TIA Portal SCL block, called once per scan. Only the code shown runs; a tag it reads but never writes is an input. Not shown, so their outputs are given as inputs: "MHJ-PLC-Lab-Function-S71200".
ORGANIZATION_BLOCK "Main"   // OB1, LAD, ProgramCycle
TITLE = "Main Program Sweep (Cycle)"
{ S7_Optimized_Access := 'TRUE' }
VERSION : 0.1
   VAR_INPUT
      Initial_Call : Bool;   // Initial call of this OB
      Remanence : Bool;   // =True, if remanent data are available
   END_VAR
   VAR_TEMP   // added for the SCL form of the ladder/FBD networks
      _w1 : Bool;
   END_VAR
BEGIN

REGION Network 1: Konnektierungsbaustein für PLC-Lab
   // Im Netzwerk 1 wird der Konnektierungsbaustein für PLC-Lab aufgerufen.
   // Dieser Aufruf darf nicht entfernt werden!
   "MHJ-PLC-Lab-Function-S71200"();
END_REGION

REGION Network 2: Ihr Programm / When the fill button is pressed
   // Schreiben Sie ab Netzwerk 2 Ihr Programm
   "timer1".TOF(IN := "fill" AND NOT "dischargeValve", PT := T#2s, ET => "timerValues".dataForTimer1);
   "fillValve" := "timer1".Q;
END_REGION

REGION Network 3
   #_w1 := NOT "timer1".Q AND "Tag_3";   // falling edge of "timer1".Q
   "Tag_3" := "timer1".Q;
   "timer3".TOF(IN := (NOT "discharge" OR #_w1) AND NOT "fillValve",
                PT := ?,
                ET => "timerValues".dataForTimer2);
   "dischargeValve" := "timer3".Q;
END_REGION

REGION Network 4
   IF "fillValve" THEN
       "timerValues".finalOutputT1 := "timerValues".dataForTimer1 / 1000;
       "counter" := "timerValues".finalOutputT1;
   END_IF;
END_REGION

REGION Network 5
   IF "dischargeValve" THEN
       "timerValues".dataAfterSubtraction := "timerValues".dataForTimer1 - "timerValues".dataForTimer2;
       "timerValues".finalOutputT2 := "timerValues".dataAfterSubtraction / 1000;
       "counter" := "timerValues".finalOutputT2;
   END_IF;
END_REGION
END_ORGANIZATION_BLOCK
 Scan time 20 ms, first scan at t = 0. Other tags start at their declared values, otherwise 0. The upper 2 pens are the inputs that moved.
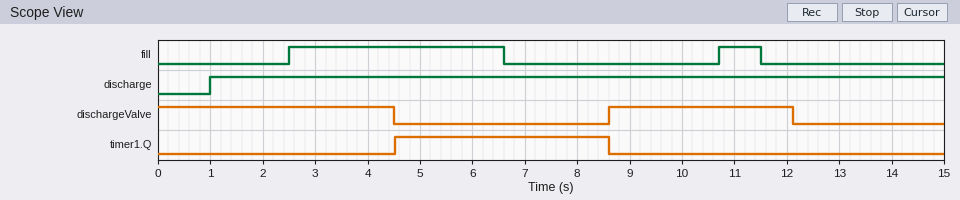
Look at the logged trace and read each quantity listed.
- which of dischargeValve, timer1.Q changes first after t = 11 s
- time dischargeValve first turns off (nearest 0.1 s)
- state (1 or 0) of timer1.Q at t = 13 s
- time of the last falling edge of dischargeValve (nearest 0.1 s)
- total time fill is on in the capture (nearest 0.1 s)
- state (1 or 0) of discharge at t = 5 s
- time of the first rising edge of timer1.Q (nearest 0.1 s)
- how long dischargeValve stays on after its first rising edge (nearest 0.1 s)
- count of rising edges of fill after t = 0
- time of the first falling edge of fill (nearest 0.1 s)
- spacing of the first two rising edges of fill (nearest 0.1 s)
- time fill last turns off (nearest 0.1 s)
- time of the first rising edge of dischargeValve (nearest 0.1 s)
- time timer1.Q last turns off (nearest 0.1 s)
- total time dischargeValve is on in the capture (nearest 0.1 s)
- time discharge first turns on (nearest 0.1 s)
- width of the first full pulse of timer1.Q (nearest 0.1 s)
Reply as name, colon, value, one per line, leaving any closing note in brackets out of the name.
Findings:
which of dischargeValve, timer1.Q changes first after t = 11 s: dischargeValve
time dischargeValve first turns off: 4.5 s
state (1 or 0) of timer1.Q at t = 13 s: 0
time of the last falling edge of dischargeValve: 12.1 s
total time fill is on in the capture: 4.9 s
state (1 or 0) of discharge at t = 5 s: 1
time of the first rising edge of timer1.Q: 4.5 s
how long dischargeValve stays on after its first rising edge: 3.5 s
count of rising edges of fill after t = 0: 2
time of the first falling edge of fill: 6.6 s
spacing of the first two rising edges of fill: 8.2 s
time fill last turns off: 11.5 s
time of the first rising edge of dischargeValve: 8.6 s
time timer1.Q last turns off: 8.6 s
total time dischargeValve is on in the capture: 8.0 s
time discharge first turns on: 1.0 s
width of the first full pulse of timer1.Q: 4.1 s
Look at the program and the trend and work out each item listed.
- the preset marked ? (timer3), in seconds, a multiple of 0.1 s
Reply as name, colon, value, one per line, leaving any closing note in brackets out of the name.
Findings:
the preset marked ? (timer3), in seconds, a multiple of 0.1 s: 3.5 s
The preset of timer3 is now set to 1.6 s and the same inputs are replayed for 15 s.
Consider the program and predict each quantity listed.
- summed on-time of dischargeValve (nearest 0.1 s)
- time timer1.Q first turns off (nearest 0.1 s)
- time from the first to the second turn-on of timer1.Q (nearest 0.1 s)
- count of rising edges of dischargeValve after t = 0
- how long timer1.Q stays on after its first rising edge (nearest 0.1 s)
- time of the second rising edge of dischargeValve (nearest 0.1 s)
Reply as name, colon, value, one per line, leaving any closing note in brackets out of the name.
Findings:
summed on-time of dischargeValve: 5.7 s
time timer1.Q first turns off: 8.6 s
time from the first to the second turn-on of timer1.Q: 8.1 s
count of rising edges of dischargeValve after t = 0: 2
how long timer1.Q stays on after its first rising edge: 6.0 s
time of the second rising edge of dischargeValve: 13.5 s
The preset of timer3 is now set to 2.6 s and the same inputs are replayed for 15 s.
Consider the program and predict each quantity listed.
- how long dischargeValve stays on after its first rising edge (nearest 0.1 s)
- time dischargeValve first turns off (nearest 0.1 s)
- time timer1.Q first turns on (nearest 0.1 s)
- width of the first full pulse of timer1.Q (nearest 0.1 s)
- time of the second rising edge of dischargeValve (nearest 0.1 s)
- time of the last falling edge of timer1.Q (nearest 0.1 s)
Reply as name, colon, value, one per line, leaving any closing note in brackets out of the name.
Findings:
how long dischargeValve stays on after its first rising edge: 2.6 s
time dischargeValve first turns off: 3.6 s
time timer1.Q first turns on: 3.6 s
width of the first full pulse of timer1.Q: 5.0 s
time of the second rising edge of dischargeValve: 13.5 s
time of the last falling edge of timer1.Q: 13.5 s
